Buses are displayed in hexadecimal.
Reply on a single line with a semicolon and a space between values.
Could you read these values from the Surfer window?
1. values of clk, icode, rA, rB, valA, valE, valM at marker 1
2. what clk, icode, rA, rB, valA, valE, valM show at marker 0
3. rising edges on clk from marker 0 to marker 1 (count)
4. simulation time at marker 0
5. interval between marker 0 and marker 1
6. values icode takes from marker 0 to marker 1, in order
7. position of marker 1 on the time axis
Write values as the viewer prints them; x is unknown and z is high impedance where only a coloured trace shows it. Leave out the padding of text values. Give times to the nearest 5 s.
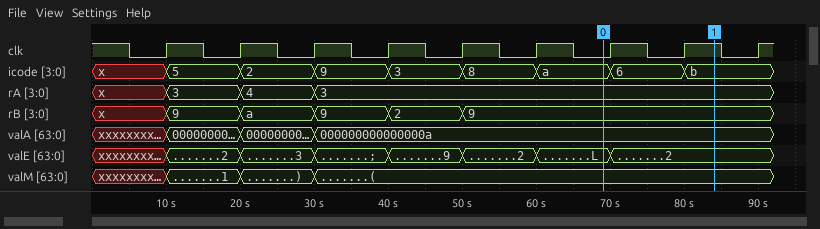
clk=1, icode=b, rA=3, rB=9, valA=000000000000000a, valE=2, valM=(; clk=0, icode=a, rA=3, rB=9, valA=000000000000000a, valE=L, valM=(; 2; 70 s; 15 s; a, 6, b; 85 s
